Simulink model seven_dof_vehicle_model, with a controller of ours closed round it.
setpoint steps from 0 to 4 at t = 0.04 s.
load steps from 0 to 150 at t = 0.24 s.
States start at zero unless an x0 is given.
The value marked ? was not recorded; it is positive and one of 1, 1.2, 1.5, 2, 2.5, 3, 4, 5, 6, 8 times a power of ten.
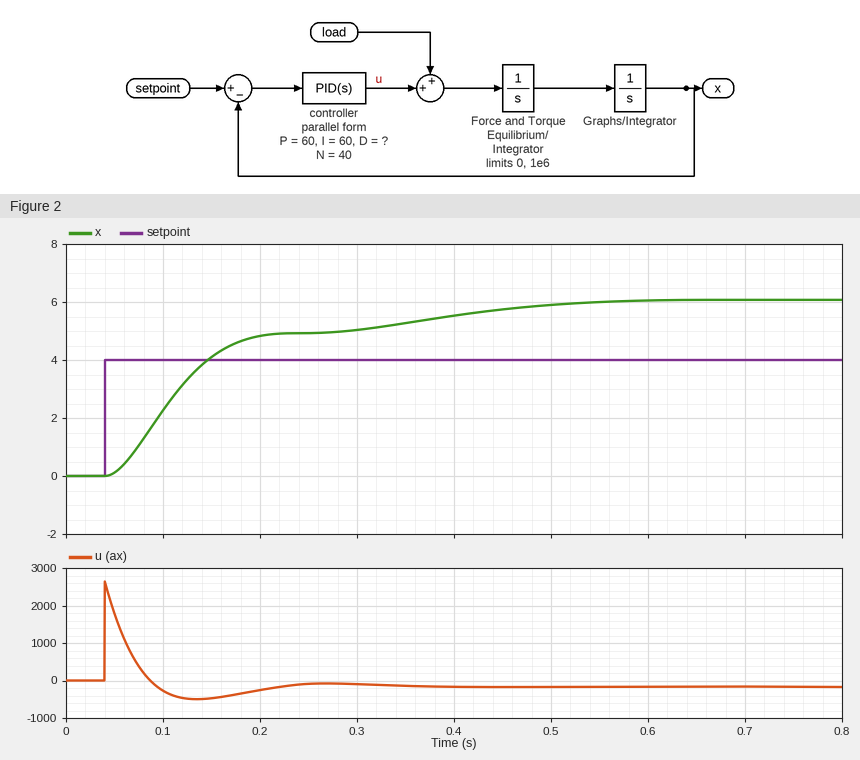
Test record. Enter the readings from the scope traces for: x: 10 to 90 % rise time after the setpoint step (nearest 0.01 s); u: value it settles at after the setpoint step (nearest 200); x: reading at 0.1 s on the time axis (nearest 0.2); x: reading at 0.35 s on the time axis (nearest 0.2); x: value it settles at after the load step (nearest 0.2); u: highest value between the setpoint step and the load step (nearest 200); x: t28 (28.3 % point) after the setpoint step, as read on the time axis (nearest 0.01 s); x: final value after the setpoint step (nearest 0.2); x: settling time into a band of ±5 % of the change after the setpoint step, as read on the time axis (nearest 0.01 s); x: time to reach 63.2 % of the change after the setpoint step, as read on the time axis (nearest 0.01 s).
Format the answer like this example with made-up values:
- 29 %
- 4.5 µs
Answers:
- 0.10 s
- -200
- 2.2
- 5.2
- 6.0
- 2600
- 0.08 s
- 5.0
- 0.18 s
- 0.12 s
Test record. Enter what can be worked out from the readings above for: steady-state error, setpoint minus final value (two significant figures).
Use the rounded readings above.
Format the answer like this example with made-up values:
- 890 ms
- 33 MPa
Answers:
- -1.0
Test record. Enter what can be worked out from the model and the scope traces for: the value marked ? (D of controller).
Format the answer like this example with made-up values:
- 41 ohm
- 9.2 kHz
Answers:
- 15
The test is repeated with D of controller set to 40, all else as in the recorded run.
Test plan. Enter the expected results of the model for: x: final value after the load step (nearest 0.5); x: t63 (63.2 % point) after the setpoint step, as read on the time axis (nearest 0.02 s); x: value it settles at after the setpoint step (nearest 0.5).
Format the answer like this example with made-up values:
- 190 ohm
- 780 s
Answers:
- 5.5
- 0.08 s
- 5.0
